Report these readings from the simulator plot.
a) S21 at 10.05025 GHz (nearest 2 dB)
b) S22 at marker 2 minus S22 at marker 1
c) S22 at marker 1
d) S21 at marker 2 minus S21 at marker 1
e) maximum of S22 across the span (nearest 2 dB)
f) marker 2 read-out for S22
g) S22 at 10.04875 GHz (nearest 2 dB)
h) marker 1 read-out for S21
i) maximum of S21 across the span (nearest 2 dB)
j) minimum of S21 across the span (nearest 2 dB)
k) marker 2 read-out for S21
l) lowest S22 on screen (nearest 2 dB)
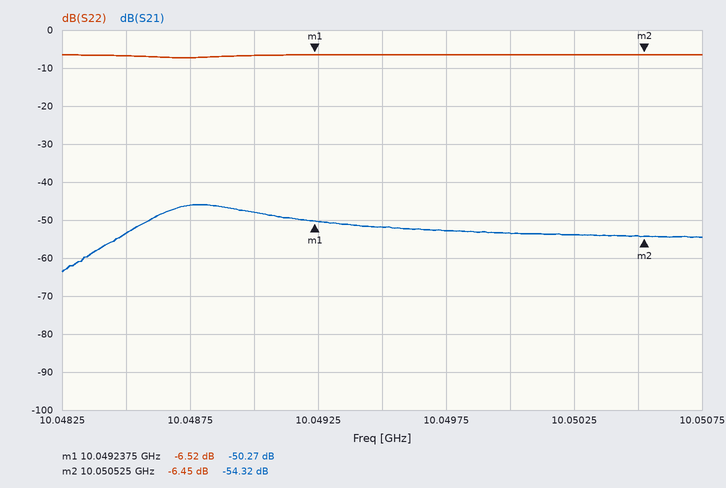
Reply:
-54 dB
0.07 dB
-6.52 dB
-4.05 dB
-6 dB
-6.45 dB
-8 dB
-50.27 dB
-46 dB
-64 dB
-54.32 dB
-8 dB
